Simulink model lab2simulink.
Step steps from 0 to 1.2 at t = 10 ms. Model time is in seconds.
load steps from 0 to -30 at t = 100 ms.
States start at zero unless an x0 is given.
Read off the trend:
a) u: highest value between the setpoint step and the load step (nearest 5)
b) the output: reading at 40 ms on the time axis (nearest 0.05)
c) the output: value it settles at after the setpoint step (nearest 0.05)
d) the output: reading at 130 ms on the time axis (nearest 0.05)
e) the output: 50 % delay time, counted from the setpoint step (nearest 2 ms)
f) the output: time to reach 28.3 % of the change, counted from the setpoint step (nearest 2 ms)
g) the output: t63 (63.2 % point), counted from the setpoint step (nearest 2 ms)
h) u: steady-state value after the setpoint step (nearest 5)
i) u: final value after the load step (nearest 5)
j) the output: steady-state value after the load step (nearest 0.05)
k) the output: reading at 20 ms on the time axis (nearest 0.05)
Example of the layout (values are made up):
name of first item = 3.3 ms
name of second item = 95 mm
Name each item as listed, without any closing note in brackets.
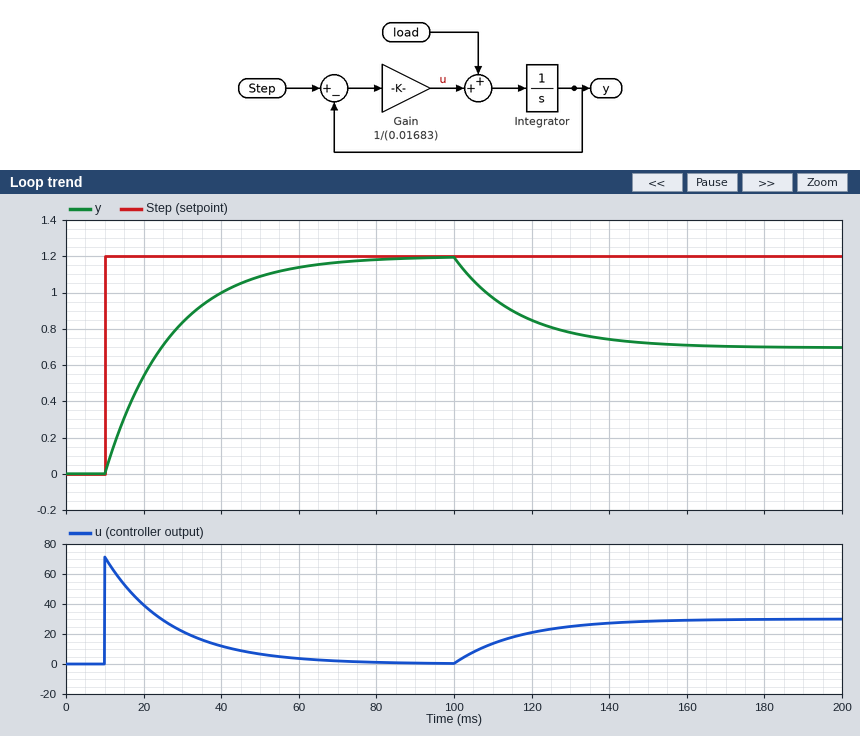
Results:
u: highest value between the setpoint step and the load step = 70
the output: reading at 40 ms on the time axis = 1.00
the output: value it settles at after the setpoint step = 1.20
the output: reading at 130 ms on the time axis = 0.80
the output: 50 % delay time, counted from the setpoint step = 12 ms
the output: time to reach 28.3 % of the change, counted from the setpoint step = 6 ms
the output: t63 (63.2 % point), counted from the setpoint step = 16 ms
u: steady-state value after the setpoint step = 0
u: final value after the load step = 30
the output: steady-state value after the load step = 0.70
the output: reading at 20 ms on the time axis = 0.55
